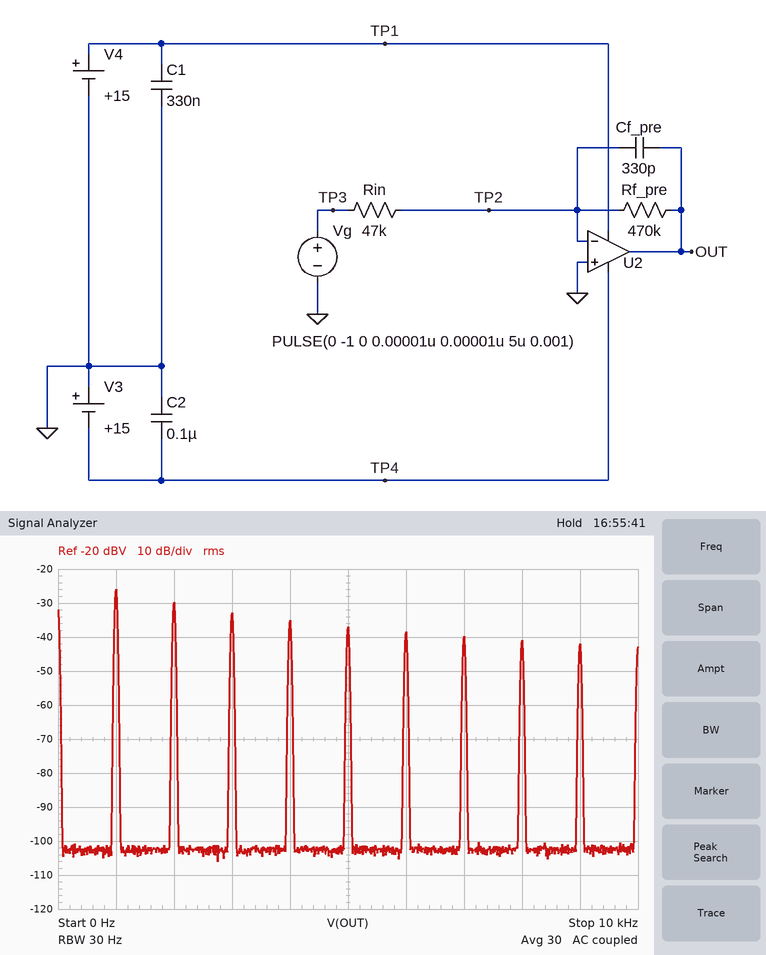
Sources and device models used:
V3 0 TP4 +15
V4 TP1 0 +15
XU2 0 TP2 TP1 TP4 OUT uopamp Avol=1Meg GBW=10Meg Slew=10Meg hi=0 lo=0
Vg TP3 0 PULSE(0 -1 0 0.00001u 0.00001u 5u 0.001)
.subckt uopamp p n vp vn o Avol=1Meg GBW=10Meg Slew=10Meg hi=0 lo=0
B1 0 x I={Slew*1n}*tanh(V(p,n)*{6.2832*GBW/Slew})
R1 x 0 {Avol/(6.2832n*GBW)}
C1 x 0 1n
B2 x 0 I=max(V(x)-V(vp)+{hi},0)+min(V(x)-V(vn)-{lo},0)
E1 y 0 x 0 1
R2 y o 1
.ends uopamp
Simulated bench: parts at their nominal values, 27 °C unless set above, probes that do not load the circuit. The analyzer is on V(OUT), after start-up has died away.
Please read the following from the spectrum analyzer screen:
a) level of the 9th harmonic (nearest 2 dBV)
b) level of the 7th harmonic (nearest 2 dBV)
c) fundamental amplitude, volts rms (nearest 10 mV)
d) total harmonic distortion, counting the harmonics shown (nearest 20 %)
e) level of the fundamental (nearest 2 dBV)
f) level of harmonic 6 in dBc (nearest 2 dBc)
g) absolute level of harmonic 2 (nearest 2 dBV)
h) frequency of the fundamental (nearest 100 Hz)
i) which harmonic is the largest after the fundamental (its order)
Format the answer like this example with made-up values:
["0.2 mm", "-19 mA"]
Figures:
["-42 dBV", "-40 dBV", "50 mV", "100 %", "-26 dBV", "-12 dBc", "-30 dBV", "1.0 kHz", "2"]
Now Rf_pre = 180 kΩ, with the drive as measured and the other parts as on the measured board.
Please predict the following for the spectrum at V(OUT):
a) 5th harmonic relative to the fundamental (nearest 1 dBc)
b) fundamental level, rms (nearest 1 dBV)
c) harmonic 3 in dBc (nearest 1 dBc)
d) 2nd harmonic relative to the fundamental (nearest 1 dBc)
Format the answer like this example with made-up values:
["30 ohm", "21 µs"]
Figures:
["-6 dBc", "-32 dBV", "-3 dBc", "-1 dBc"]
